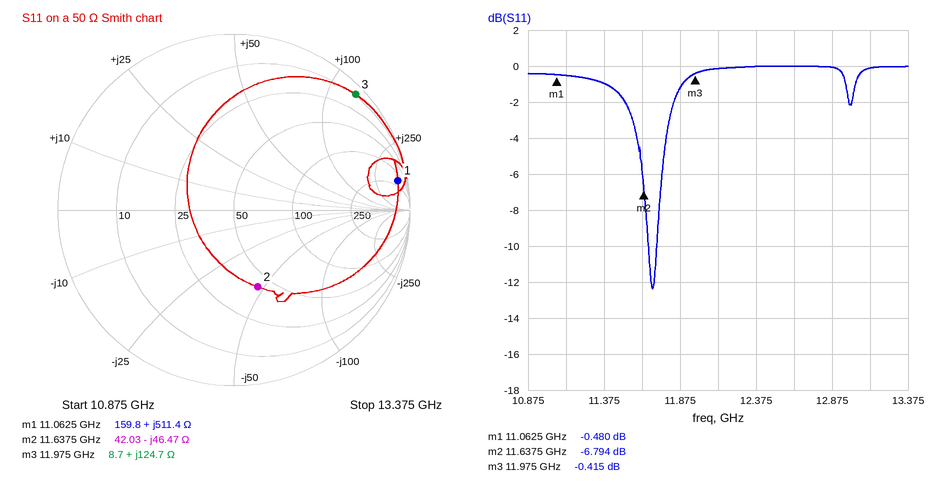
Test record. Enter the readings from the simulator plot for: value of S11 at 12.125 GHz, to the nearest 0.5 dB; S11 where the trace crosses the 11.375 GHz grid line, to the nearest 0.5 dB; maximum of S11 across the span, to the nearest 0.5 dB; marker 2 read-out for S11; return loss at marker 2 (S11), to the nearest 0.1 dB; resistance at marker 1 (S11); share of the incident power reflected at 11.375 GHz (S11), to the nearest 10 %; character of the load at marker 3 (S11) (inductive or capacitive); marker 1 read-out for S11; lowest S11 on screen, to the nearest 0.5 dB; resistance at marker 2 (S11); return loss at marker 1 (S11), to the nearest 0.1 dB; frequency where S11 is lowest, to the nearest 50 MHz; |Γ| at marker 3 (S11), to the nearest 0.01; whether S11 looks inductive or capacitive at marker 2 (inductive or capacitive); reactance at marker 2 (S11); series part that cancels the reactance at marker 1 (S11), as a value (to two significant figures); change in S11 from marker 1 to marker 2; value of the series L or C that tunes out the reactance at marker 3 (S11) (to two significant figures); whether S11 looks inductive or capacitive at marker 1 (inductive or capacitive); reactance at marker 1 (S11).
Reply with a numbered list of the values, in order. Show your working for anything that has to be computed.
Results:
1. 0.0 dB
2. -1.0 dB
3. 0.0 dB
4. -6.794 dB
5. 6.8 dB
6. 159.8 Ω
7. 10^(-1/10) ≈ 79.4 %, so 80 % to the nearest 10 %
8. inductive
9. -0.480 dB
10. -12.5 dB
11. 42.03 Ω
12. 0.5 dB
13. 11.70 GHz
14. 0.95
15. capacitive
16. -46.47 Ω
17. C = 1/(2π × 11.0625 GHz × 511.4 Ω) ≈ 28 fF
18. -6.794 − (-0.48) = -6.314 dB
19. C = 1/(2π × 11.975 GHz × 124.7 Ω) ≈ 107 fF, so 110 fF to two significant figures
20. inductive
21. +511.4 Ω
